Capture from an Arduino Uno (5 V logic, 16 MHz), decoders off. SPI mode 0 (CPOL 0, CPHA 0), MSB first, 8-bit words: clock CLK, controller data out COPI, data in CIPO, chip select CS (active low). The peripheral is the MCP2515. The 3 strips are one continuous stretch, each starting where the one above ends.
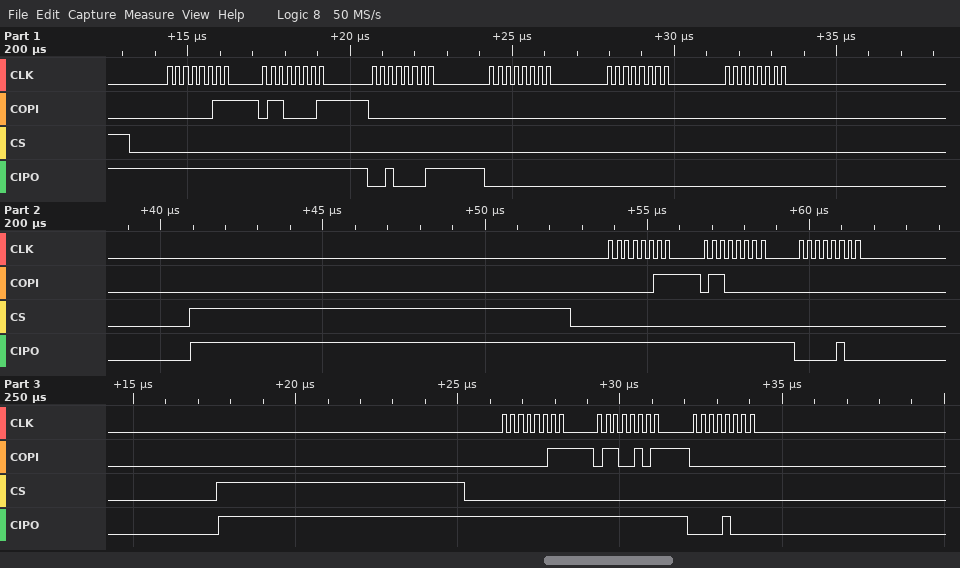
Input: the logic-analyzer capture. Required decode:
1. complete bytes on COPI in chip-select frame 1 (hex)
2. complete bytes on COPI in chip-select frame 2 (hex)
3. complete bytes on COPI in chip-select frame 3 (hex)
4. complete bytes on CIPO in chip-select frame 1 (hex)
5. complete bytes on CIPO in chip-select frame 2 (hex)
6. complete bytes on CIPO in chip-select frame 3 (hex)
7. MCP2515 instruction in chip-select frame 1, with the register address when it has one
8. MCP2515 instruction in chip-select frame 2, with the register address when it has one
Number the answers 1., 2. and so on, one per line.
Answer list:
1. 03 61 00 00 00 00
2. 03 60 00
3. 03 65 00
4. FF FF 21 00 00 00
5. FF FF 04
6. FF FF 08
7. READ 0x61
8. READ 0x60
